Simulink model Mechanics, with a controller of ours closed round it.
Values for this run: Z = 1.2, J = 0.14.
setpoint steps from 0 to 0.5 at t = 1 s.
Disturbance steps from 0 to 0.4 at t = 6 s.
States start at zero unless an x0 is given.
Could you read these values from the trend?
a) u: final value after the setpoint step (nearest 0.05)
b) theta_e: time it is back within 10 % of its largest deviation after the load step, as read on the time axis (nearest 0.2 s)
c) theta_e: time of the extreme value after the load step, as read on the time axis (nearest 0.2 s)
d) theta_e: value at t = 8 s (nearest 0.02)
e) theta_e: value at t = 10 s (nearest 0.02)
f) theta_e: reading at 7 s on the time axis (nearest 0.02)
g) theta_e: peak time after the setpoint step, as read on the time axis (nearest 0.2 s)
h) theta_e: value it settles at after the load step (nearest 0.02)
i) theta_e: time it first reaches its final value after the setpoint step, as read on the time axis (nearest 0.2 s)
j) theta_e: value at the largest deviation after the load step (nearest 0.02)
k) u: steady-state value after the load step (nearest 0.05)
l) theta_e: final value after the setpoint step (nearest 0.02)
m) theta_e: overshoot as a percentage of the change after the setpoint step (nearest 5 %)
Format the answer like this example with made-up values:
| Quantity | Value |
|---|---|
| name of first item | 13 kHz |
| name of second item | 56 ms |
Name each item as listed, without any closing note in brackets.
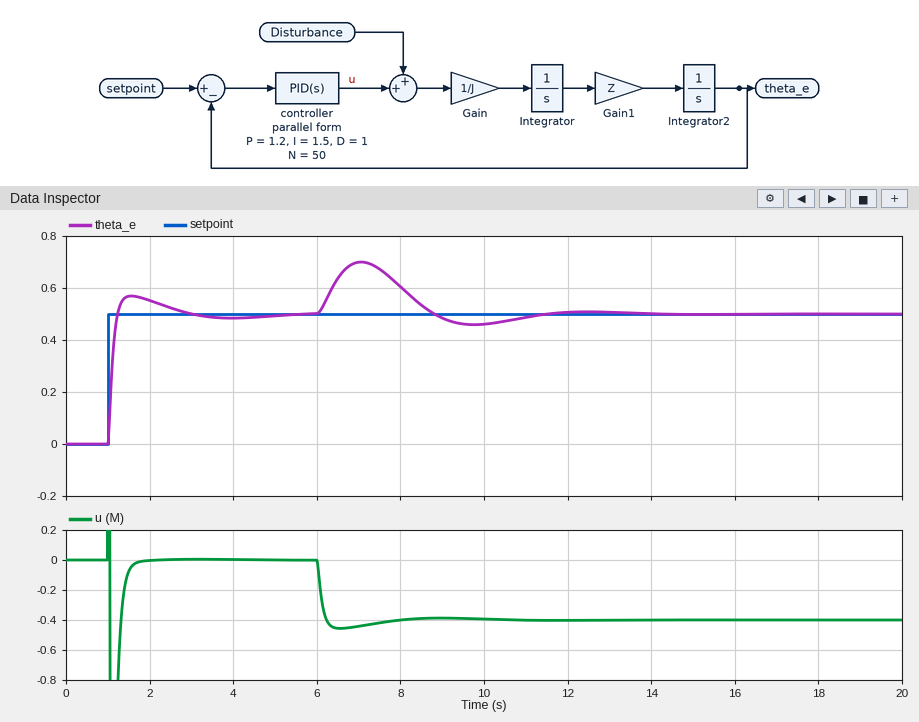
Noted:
| Quantity | Value |
|---|---|
| u: final value after the setpoint step | 0.00 |
| theta_e: time it is back within 10 % of its largest deviation after the load step, as read on the time axis | 10.8 s |
| theta_e: time of the extreme value after the load step, as read on the time axis | 7.0 s |
| theta_e: value at t = 8 s | 0.60 |
| theta_e: value at t = 10 s | 0.46 |
| theta_e: reading at 7 s on the time axis | 0.70 |
| theta_e: peak time after the setpoint step, as read on the time axis | 1.6 s |
| theta_e: value it settles at after the load step | 0.50 |
| theta_e: time it first reaches its final value after the setpoint step, as read on the time axis | 1.2 s |
| theta_e: value at the largest deviation after the load step | 0.70 |
| u: steady-state value after the load step | -0.40 |
| theta_e: final value after the setpoint step | 0.50 |
| theta_e: overshoot as a percentage of the change after the setpoint step | 15 % |
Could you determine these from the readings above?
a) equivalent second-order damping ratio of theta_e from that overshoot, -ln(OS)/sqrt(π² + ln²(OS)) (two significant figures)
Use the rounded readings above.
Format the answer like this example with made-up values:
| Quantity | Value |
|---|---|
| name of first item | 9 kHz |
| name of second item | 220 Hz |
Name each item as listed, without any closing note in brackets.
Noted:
| Quantity | Value |
|---|---|
| equivalent second-order damping ratio of theta_e from that overshoot, -ln(OS)/sqrt(π² + ln²(OS)) | 0.52 |
